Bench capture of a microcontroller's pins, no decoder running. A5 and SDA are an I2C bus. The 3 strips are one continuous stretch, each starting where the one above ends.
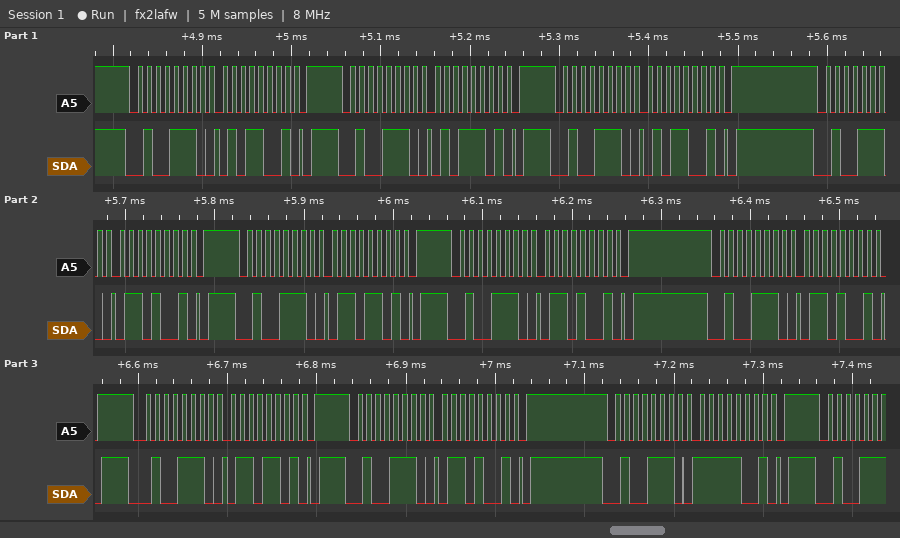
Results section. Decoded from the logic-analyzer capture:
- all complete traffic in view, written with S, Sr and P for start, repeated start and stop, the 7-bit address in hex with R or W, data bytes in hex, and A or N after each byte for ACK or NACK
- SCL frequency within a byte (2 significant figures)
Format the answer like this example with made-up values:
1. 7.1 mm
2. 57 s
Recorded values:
1. S 27W A 59 A P S 27W A 5D A P S 27W A 59 A P S 27W A 69 A P S 27W A 6D A P S 27W A 69 A P S 27W A 69 A P S 27W A 6D A P S 27W A 69 A P S 27W A F9 A P
2. 100 kHz
